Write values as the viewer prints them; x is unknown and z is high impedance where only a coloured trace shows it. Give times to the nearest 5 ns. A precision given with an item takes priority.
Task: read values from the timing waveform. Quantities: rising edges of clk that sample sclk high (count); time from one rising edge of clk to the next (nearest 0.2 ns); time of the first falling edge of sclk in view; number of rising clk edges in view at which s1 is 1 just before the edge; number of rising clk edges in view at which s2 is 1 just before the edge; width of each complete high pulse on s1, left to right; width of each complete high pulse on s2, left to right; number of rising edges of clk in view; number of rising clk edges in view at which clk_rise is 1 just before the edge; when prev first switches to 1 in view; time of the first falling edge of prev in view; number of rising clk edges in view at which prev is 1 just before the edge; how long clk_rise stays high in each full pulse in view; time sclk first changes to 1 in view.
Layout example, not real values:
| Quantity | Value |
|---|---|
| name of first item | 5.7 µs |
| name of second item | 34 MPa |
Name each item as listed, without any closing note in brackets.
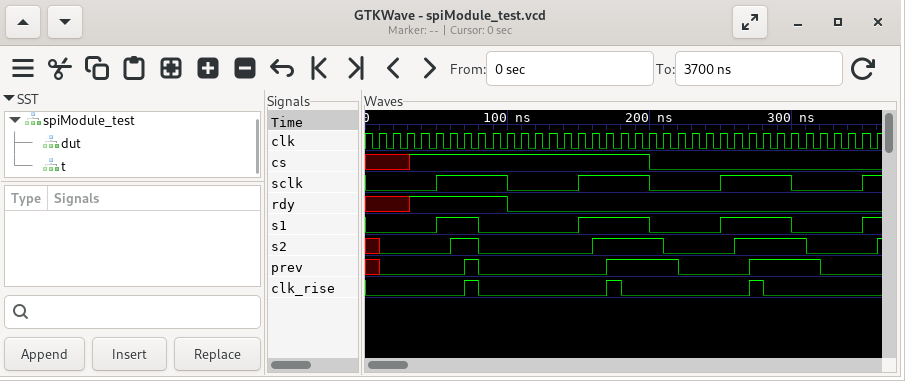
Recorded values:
| Quantity | Value |
|---|---|
| rising edges of clk that sample sclk high | 16 |
| time from one rising edge of clk to the next | 10 ns |
| time of the first falling edge of sclk in view | 100 ns |
| number of rising clk edges in view at which s1 is 1 just before the edge | 14 |
| number of rising clk edges in view at which s2 is 1 just before the edge | 12 |
| width of each complete high pulse on s1, left to right | 30 ns, 50 ns, 50 ns |
| width of each complete high pulse on s2, left to right | 20 ns, 50 ns, 50 ns |
| number of rising edges of clk in view | 36 |
| number of rising clk edges in view at which clk_rise is 1 just before the edge | 3 |
| when prev first switches to 1 in view | 70 ns |
| time of the first falling edge of prev in view | 80 ns |
| number of rising clk edges in view at which prev is 1 just before the edge | 11 |
| how long clk_rise stays high in each full pulse in view | 10 ns, 10 ns, 10 ns |
| time sclk first changes to 1 in view | 50 ns |
